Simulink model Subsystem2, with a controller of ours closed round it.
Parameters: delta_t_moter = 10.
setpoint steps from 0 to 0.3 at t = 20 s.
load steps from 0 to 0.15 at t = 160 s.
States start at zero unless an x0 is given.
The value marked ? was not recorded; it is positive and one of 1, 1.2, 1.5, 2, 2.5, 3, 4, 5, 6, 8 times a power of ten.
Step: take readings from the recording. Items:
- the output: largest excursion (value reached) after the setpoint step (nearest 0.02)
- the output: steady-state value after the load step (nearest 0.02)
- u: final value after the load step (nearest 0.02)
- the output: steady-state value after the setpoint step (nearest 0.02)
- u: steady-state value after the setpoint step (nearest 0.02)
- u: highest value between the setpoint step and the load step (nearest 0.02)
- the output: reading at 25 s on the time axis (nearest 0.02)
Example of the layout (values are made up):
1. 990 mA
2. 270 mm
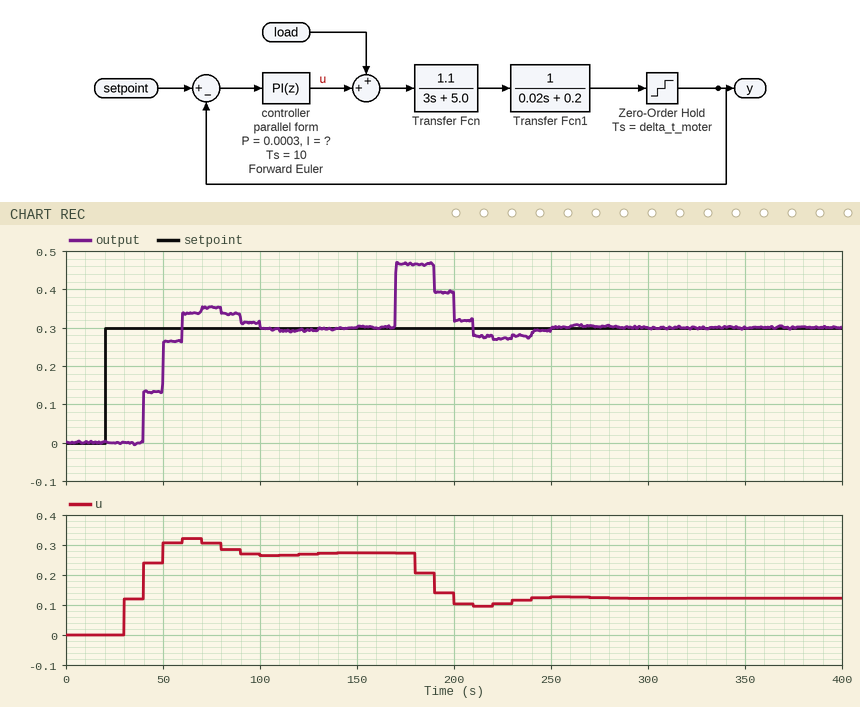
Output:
1. 0.36
2. 0.30
3. 0.12
4. 0.30
5. 0.28
6. 0.32
7. 0.00
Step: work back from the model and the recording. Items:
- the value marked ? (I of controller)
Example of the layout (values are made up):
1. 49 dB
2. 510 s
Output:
1. 0.04
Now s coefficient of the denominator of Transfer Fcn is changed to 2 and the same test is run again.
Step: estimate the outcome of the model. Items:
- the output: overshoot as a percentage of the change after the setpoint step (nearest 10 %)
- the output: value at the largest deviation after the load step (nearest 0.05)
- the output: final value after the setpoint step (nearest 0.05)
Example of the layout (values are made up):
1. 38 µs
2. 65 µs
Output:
1. 20 %
2. 0.45
3. 0.30
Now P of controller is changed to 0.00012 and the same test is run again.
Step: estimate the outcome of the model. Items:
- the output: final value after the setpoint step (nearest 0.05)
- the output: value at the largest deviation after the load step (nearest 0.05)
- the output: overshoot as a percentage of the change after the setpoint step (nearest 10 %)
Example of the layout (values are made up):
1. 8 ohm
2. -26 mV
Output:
1. 0.30
2. 0.45
3. 20 %
